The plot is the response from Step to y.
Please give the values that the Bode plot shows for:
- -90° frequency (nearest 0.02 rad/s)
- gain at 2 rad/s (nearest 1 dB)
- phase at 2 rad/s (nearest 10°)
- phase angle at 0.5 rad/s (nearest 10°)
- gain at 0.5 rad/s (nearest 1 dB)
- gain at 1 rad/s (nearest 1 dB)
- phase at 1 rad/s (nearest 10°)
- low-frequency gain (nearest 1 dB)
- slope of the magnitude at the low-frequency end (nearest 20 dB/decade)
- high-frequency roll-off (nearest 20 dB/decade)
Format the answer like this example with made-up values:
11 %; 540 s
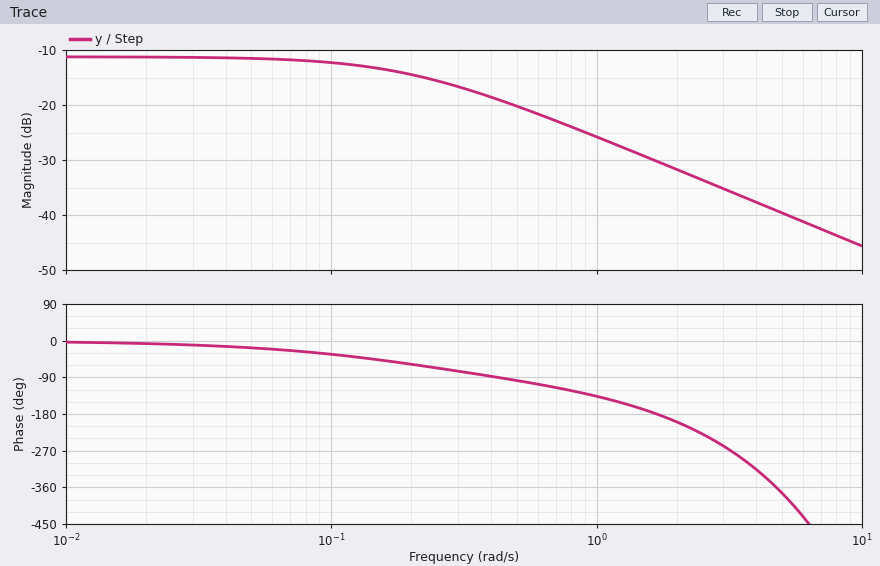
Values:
0.42 rad/s; -32 dB; -200°; -100°; -20 dB; -26 dB; -140°; -11 dB; 0 dB/decade; -20 dB/decade
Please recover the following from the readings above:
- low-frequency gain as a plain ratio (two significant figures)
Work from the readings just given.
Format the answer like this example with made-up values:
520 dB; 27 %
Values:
0.28
